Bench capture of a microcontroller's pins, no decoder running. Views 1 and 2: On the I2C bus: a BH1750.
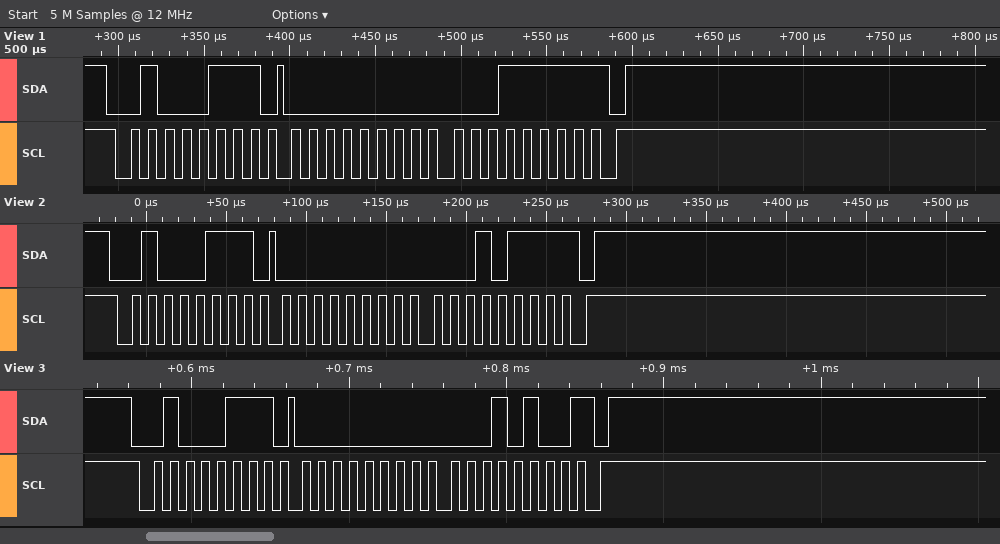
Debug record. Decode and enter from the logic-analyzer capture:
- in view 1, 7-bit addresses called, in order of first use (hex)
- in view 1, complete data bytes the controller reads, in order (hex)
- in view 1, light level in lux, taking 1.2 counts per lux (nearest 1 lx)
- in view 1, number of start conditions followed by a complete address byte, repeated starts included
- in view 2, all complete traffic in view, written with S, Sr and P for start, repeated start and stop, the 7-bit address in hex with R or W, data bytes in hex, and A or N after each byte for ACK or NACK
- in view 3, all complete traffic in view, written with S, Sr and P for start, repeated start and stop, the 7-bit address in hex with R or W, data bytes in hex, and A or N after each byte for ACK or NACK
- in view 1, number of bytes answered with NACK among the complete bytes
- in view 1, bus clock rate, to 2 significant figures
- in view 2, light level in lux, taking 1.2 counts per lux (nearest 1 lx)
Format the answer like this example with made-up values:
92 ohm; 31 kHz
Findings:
0x23; 00 1F; 26 lx; 1; S 23R A 00 A 17 N P; S 23R A 00 A 14 N P; 1; 100 kHz; 19 lx
